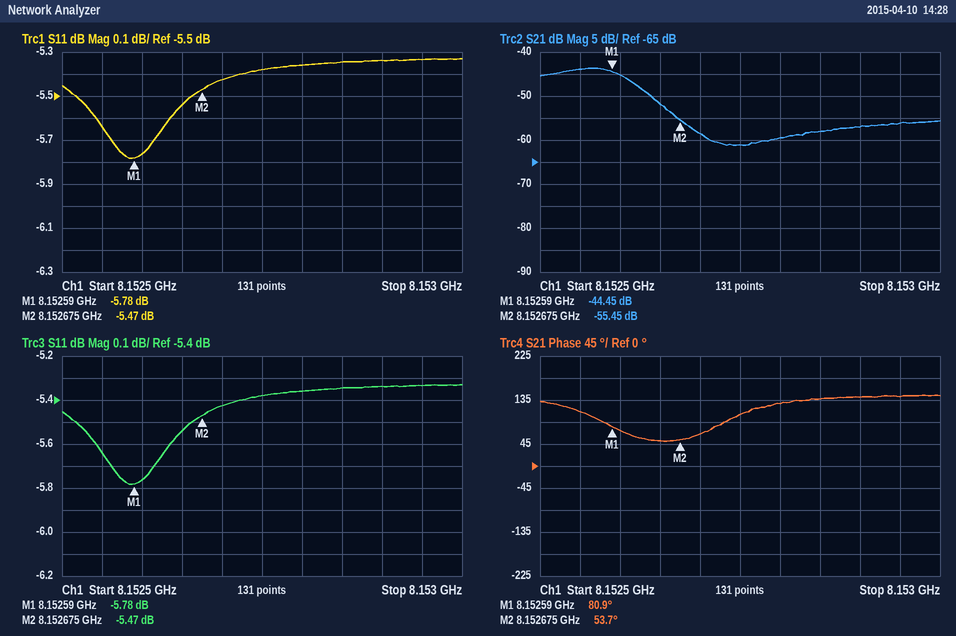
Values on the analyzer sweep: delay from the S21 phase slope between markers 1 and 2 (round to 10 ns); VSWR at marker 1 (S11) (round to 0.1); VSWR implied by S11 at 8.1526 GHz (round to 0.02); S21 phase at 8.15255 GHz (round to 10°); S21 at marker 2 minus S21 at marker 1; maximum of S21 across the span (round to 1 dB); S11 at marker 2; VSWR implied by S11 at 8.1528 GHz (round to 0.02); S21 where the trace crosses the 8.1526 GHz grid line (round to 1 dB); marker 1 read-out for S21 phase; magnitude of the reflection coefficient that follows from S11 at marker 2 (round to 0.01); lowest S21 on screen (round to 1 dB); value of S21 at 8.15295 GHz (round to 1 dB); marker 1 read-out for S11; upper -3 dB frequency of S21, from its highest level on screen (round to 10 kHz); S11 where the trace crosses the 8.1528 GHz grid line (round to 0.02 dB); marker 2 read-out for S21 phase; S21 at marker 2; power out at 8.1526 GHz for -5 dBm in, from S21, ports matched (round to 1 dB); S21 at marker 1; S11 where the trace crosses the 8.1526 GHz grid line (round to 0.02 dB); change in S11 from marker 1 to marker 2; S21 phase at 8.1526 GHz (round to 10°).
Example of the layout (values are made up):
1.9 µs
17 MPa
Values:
890 ns
3.1
3.12
110°
-11.00 dB
-44 dB
-5.47 dB
3.34
-45 dB
80.9°
0.53
-61 dB
-56 dB
-5.78 dB
8.15261 GHz
-5.36 dB
53.7°
-55.45 dB
-50 dBm
-44.45 dB
-5.76 dB
0.31 dB
70°
